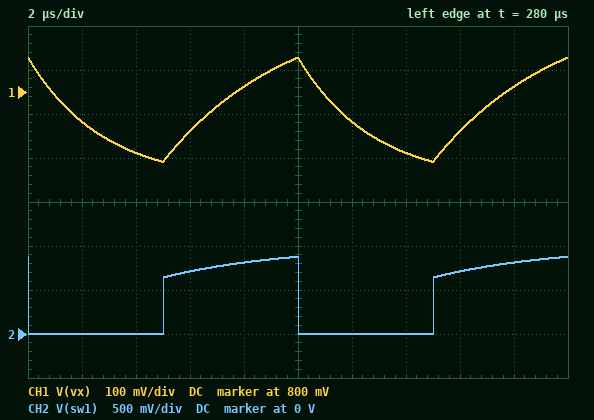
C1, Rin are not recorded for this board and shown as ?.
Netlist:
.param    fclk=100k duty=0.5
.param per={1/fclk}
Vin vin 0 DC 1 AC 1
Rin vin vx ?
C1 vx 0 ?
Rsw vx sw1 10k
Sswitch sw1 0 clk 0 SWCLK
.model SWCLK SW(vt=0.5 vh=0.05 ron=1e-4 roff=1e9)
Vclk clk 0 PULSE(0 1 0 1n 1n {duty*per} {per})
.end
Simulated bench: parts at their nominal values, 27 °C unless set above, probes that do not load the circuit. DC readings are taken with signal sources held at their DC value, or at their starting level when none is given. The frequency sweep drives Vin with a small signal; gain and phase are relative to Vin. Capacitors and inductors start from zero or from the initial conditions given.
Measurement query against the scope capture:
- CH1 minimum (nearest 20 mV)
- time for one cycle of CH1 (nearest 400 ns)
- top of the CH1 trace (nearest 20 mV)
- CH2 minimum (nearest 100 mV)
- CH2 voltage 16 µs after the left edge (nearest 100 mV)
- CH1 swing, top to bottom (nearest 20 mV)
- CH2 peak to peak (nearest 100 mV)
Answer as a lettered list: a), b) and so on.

a) 640 mV
b) 10.0 µs
c) 880 mV
d) 0 V
e) 700 mV
f) 240 mV
g) 900 mV
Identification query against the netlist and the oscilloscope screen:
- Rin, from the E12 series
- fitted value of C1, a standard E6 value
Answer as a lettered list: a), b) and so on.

a) 6.8 kΩ
b) 680 pF
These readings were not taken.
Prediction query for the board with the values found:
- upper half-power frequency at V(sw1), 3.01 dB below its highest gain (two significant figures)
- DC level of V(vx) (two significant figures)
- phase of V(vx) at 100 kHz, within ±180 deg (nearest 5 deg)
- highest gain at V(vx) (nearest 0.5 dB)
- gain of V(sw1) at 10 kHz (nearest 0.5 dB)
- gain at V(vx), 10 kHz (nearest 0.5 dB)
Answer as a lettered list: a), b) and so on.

a) 34 kHz
b) 1.0 V
c) -70 deg
d) 0 dB
e) -0.5 dB
f) -0.5 dB
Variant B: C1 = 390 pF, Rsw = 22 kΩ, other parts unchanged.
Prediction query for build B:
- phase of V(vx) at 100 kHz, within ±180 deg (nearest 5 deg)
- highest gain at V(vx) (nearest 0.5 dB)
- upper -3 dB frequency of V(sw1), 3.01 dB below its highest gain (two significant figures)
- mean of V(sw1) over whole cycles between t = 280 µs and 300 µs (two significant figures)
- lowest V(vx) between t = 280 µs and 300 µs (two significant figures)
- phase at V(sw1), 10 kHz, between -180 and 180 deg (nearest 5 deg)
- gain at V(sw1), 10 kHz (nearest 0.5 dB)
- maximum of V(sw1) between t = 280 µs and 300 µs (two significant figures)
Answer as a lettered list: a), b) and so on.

a) -60 deg
b) 0 dB
c) 60 kHz
d) 450 mV
e) 780 mV
f) -10 deg
g) 0 dB
h) 970 mV
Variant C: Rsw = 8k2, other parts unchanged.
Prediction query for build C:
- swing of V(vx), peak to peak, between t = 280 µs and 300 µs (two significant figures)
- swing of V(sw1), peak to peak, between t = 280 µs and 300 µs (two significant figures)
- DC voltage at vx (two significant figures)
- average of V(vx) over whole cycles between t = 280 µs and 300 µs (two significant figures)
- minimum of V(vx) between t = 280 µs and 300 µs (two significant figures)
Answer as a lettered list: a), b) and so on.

a) 270 mV
b) 860 mV
c) 1.0 V
d) 720 mV
e) 590 mV
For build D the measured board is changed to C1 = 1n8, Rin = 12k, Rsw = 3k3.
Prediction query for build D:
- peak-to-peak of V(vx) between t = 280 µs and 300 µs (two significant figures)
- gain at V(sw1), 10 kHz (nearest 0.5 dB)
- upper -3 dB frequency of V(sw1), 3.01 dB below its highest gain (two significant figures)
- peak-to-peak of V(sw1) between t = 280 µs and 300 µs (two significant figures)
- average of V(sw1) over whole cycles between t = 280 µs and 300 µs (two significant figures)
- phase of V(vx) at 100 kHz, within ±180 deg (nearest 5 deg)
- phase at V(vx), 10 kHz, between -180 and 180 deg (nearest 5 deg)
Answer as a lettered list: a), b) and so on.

a) 150 mV
b) -4.5 dB
c) 7.4 kHz
d) 440 mV
e) 180 mV
f) -85 deg
g) -55 deg
